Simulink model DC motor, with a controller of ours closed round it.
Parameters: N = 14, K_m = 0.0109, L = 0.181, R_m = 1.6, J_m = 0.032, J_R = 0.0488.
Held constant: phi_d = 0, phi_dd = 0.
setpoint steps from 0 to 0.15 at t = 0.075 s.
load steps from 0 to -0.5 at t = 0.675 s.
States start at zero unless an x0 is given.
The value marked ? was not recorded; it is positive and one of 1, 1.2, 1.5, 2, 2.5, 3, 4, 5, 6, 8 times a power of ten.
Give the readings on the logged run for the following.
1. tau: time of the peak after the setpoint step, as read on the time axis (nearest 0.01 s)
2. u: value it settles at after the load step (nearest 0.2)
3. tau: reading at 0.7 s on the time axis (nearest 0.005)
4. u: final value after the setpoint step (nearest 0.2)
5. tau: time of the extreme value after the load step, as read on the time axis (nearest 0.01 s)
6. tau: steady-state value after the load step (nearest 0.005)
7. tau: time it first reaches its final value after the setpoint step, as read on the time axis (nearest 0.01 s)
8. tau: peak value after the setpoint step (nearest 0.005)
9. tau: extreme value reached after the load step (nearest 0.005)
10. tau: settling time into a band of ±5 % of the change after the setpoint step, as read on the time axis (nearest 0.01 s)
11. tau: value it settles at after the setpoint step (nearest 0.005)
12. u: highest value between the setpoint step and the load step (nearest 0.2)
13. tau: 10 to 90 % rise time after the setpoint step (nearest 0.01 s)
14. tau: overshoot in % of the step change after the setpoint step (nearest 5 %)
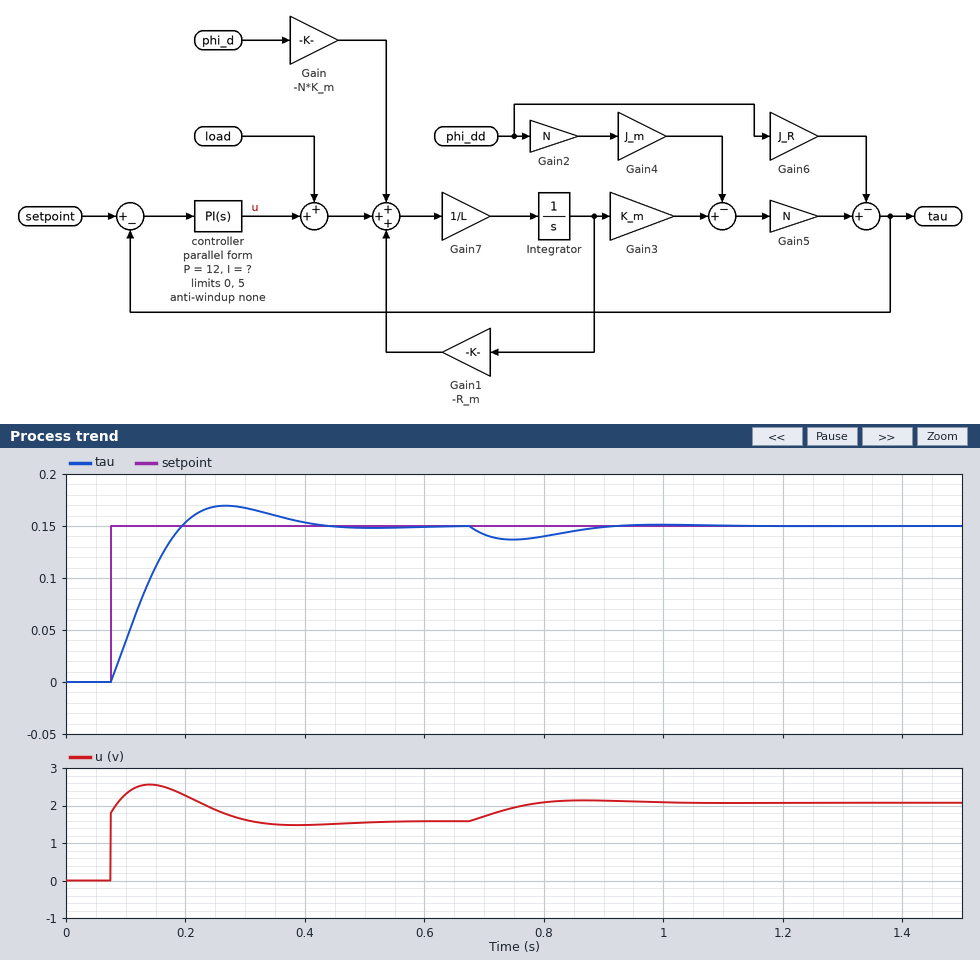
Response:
0.27 s
2.0
0.140
1.6
0.75 s
0.150
0.19 s
0.170
0.135
0.37 s
0.150
2.6
0.09 s
15 %
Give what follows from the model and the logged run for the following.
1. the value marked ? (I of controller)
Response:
300
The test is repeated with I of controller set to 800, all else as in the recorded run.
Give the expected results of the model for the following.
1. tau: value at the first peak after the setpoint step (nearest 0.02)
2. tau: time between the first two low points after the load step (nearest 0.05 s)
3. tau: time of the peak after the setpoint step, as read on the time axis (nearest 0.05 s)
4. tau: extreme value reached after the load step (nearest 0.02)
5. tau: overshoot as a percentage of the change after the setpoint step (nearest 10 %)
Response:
0.20
0.25 s
0.20 s
0.14
30 %
